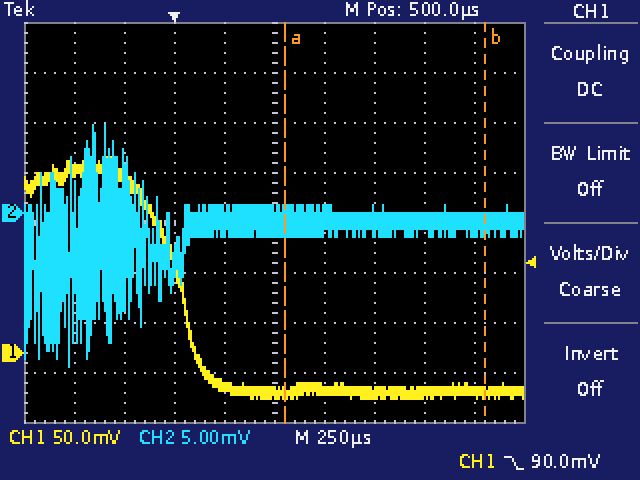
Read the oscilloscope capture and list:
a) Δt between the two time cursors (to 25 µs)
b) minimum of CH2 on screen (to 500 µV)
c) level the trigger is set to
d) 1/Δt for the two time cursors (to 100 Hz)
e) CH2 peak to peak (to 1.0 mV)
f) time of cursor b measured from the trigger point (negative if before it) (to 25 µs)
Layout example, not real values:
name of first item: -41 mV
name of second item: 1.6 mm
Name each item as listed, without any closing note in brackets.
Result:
Δt between the two time cursors: 1.000 ms
minimum of CH2 on screen: -15.5 mV
level the trigger is set to: 90.0 mV
1/Δt for the two time cursors: 1.0 kHz
CH2 peak to peak: 24.0 mV
time of cursor b measured from the trigger point (negative if before it): +1.550 ms
